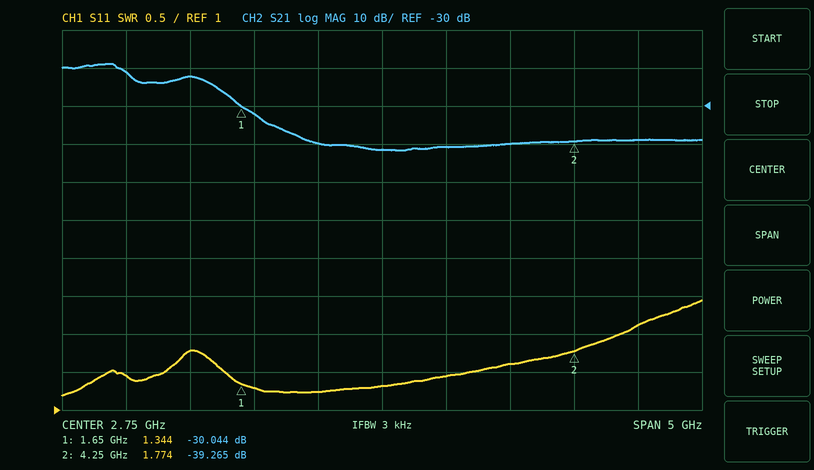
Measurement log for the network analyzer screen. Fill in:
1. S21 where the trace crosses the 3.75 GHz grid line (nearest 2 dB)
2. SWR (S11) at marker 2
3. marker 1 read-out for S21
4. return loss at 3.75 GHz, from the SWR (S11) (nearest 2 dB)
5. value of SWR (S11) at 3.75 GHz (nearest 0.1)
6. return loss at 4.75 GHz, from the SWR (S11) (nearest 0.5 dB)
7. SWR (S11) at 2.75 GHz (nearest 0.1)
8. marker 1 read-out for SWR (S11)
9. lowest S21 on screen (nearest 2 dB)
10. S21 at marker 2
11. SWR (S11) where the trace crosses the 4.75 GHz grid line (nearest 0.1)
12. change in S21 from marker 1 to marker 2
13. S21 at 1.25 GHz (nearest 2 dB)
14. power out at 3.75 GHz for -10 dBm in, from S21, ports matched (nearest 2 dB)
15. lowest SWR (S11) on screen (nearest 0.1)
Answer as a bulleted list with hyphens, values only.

- -40 dB
- 1.774
- -30.044 dB
- 12 dB
- 1.6
- 9.0 dB
- 1.3
- 1.344
- -42 dB
- -39.265 dB
- 2.1
- -9.221 dB
- -22 dB
- -50 dBm
- 1.2
